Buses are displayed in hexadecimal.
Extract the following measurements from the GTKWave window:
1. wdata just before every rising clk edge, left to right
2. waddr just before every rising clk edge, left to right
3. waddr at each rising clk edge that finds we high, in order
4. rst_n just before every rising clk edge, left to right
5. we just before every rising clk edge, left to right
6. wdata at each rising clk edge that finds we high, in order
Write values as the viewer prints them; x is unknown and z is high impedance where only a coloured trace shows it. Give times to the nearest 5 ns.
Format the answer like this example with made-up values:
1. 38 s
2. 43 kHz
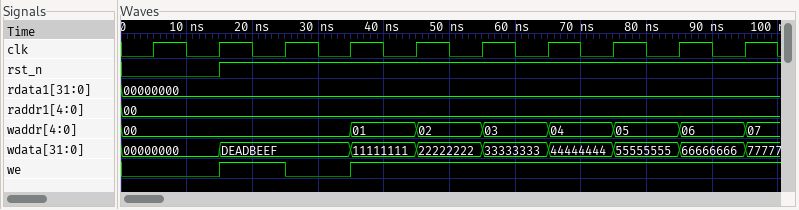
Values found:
1. 00000000, 00000000, DEADBEEF, DEADBEEF, 11111111, 22222222, 33333333, 44444444, 55555555, 66666666
2. 00, 00, 00, 00, 01, 02, 03, 04, 05, 06
3. 00, 01, 02, 03, 04, 05, 06
4. 0 0 1 1 1 1 1 1 1 1
5. 0 0 1 0 1 1 1 1 1 1
6. DEADBEEF, 11111111, 22222222, 33333333, 44444444, 55555555, 66666666
